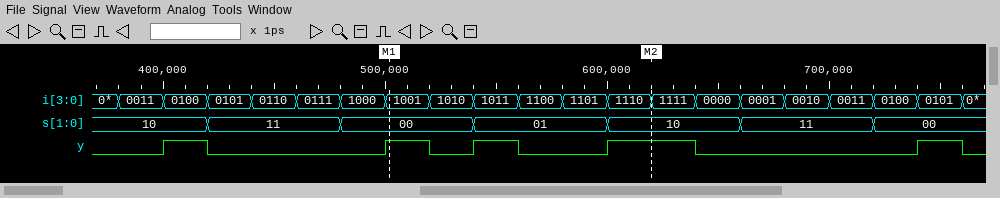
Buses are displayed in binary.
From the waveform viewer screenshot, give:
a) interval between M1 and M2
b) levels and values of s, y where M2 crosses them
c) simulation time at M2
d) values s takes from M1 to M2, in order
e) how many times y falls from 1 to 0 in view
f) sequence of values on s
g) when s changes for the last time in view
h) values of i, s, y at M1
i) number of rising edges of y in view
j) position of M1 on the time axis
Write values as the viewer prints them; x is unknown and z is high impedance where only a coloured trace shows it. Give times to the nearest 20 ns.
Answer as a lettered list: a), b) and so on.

a) 120 ns
b) s=10, y=1
c) 620 ns
d) 00, 01, 10
e) 5
f) 10, 11, 00, 01, 10, 11, 00
g) 720 ns
h) i=1001, s=00, y=1
i) 5
j) 500 ns
